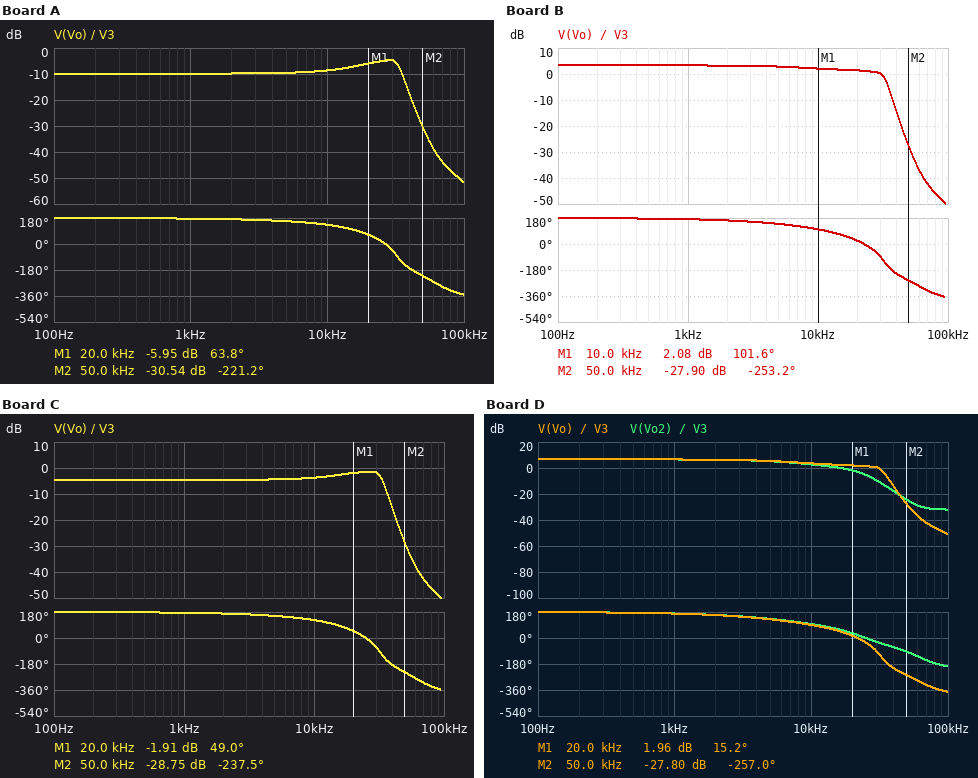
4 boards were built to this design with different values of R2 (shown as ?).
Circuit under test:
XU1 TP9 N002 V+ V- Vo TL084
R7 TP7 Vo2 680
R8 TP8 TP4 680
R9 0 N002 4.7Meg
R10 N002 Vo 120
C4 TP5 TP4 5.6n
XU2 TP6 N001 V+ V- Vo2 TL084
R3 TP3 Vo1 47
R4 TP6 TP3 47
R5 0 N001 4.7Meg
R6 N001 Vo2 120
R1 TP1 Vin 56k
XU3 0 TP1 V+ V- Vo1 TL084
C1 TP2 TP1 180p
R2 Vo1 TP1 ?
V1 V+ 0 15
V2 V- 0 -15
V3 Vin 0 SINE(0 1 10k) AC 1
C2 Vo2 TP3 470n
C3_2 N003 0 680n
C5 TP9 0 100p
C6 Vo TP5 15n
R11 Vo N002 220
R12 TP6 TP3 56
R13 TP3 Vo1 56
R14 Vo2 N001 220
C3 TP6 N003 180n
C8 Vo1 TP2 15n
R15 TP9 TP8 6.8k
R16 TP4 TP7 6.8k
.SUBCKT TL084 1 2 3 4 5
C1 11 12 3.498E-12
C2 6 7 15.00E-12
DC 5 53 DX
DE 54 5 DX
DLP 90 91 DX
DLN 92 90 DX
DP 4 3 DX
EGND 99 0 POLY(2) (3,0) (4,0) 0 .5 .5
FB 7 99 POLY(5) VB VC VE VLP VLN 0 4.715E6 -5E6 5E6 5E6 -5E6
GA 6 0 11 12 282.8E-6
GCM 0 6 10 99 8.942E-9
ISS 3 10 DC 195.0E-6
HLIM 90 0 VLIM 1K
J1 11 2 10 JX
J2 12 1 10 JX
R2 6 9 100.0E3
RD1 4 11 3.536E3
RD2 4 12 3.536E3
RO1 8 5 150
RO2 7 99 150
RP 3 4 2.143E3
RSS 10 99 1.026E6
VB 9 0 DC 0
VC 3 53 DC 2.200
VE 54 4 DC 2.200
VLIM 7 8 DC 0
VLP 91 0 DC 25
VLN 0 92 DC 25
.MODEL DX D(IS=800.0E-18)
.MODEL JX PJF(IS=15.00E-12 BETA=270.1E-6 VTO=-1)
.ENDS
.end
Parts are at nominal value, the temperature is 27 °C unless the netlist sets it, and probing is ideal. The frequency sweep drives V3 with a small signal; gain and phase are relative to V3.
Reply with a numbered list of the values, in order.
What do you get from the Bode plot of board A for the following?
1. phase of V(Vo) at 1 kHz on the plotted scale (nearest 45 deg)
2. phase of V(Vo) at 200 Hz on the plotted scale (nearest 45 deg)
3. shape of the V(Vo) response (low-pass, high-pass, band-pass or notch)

1. 180 deg
2. 180 deg
3. low-pass
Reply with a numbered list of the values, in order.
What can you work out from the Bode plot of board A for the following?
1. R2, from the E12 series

1. 18 kΩ
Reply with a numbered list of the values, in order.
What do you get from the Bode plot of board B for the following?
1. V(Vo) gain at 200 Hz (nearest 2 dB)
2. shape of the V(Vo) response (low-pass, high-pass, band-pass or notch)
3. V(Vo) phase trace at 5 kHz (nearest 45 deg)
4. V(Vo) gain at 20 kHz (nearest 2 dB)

1. 4 dB
2. low-pass
3. 135 deg
4. 2 dB
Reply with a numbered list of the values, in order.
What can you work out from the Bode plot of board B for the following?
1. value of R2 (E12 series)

1. 82 kΩ
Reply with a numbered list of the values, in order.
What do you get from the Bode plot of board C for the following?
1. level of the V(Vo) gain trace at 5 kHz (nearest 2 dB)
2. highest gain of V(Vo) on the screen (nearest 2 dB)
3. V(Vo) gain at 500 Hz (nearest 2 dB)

1. -4 dB
2. -2 dB
3. -4 dB
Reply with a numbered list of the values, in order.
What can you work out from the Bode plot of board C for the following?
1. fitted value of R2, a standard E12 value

1. 33 kΩ
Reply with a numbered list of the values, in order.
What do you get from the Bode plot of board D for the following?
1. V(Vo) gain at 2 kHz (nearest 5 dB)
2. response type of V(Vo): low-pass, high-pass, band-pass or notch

1. 5 dB
2. low-pass
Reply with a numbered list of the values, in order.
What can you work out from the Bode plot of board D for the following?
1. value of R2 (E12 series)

1. 120 kΩ
